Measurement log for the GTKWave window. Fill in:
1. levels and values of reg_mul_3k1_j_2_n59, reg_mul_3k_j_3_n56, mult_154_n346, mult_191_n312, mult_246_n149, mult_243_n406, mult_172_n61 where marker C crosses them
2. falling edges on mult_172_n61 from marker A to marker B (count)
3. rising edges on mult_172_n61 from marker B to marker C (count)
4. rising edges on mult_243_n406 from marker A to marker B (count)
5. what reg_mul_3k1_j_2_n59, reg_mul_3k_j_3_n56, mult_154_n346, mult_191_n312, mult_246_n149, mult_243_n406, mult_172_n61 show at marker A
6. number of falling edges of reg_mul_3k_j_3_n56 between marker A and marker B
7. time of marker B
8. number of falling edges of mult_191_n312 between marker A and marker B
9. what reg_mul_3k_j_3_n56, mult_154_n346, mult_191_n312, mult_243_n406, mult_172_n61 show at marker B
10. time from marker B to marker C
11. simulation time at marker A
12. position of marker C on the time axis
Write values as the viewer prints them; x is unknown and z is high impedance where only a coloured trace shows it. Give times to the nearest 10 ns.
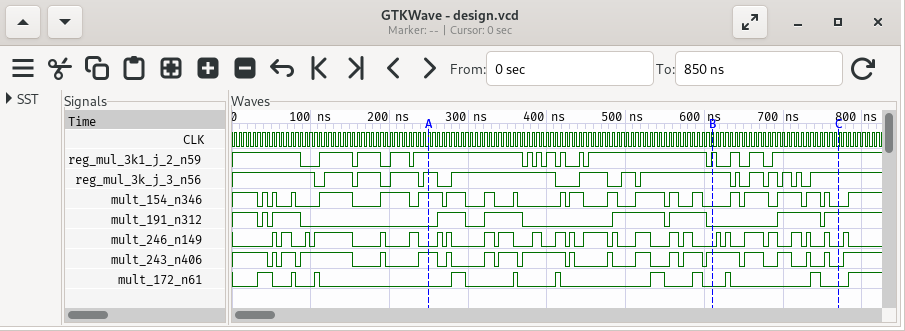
reg_mul_3k1_j_2_n59=1, reg_mul_3k_j_3_n56=1, mult_154_n346=0, mult_191_n312=1, mult_246_n149=0, mult_243_n406=0, mult_172_n61=0
5
2
10
reg_mul_3k1_j_2_n59=1, reg_mul_3k_j_3_n56=1, mult_154_n346=1, mult_191_n312=0, mult_246_n149=0, mult_243_n406=1, mult_172_n61=0
4
610 ns
4
reg_mul_3k_j_3_n56=1, mult_154_n346=0, mult_191_n312=0, mult_243_n406=1, mult_172_n61=0
160 ns
250 ns
770 ns
